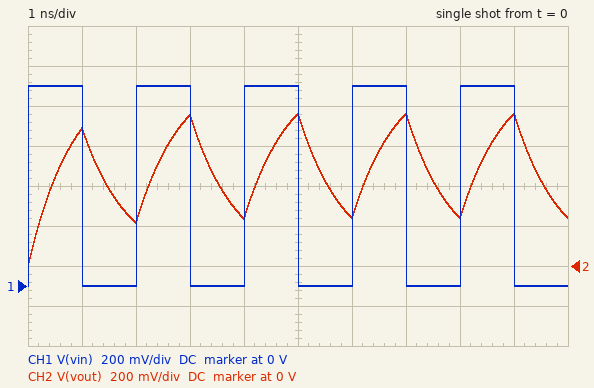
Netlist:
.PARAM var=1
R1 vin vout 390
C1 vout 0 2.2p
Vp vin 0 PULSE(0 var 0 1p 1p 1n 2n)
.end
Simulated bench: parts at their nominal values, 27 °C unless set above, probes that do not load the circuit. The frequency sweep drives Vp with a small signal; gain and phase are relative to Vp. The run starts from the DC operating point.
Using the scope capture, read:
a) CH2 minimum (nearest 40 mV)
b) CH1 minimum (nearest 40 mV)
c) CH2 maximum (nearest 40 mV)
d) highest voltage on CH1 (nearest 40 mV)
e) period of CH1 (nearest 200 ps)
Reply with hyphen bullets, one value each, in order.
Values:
- 0 V
- 0 V
- 760 mV
- 1.00 V
- 2.0 ns
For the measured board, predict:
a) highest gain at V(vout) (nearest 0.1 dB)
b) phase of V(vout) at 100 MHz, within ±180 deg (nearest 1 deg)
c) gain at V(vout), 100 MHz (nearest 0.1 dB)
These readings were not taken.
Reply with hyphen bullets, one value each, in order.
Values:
- 0 dB
- -28 deg
- -1.1 dB
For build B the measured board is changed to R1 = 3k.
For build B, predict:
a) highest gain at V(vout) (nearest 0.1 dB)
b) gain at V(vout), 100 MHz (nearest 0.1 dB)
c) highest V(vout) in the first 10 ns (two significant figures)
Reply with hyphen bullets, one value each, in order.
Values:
- 0 dB
- -12.6 dB
- 420 mV
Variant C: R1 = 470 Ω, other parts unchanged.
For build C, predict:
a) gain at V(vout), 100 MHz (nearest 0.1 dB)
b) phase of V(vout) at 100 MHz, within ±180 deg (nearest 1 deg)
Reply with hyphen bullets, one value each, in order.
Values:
- -1.5 dB
- -33 deg
